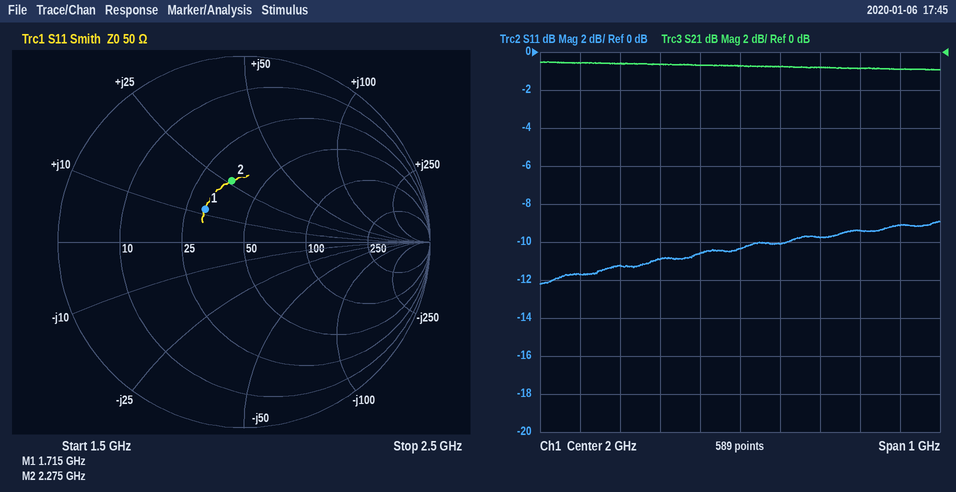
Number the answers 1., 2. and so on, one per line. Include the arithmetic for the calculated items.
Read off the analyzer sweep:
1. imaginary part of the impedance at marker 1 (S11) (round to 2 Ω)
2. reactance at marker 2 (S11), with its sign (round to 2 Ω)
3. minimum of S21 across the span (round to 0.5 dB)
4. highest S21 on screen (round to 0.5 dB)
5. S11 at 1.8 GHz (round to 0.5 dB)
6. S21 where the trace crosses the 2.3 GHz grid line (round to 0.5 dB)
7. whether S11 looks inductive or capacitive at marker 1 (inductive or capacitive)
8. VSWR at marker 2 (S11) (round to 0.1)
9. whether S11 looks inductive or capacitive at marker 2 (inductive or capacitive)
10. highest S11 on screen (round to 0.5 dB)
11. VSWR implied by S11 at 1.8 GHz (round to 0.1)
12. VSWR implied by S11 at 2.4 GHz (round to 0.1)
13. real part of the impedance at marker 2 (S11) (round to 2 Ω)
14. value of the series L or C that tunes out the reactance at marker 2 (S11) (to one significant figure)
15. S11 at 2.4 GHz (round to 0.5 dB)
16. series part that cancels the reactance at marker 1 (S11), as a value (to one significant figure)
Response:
1. +12 Ω
2. +26 Ω
3. -1.0 dB
4. -0.5 dB
5. -11.0 dB
6. -1.0 dB
7. inductive
8. 2.0
9. inductive
10. -9.0 dB
11. |Γ| = 10^(-11/20) = 0.2818; VSWR = (1 + 0.2818)/(1 − 0.2818) ≈ 1.8
12. |Γ| = 10^(-9/20) = 0.3548; VSWR = (1 + 0.3548)/(1 − 0.3548) ≈ 2.1
13. 36 Ω
14. C = 1/(2π × 2.275 GHz × 26 Ω) ≈ 3 pF
15. -9.0 dB
16. C = 1/(2π × 1.715 GHz × 12 Ω) ≈ 8 pF
